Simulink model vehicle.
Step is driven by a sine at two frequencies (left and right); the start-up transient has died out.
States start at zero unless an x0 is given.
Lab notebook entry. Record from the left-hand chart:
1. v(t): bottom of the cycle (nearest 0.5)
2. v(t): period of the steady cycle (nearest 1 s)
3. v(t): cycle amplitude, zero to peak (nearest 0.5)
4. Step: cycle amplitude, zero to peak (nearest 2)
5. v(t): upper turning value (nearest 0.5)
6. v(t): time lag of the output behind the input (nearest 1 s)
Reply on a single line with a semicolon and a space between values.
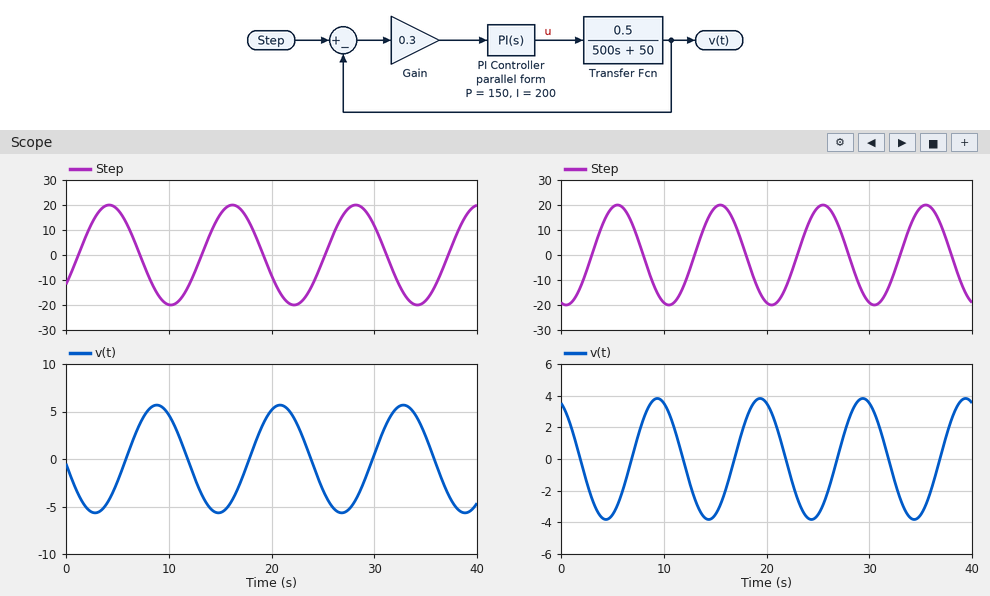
-5.5; 12 s; 5.5; 20; 5.5; 5 s
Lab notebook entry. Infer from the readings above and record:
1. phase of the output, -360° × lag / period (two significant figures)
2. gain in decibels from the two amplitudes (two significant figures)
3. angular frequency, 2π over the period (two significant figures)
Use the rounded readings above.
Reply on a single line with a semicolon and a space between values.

-150°; -11 dB; 0.52 rad/s
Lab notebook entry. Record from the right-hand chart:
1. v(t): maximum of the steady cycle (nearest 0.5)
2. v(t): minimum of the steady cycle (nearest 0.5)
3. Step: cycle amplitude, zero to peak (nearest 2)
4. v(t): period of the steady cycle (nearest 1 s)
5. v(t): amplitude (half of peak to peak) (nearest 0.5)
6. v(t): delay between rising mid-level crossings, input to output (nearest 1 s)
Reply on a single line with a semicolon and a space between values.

4.0; -4.0; 20; 10 s; 4.0; 4 s
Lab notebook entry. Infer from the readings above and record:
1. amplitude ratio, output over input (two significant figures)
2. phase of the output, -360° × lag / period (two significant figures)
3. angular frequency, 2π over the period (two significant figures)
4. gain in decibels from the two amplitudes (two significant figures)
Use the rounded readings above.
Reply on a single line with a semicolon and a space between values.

0.20; -140°; 0.63 rad/s; -14 dB
